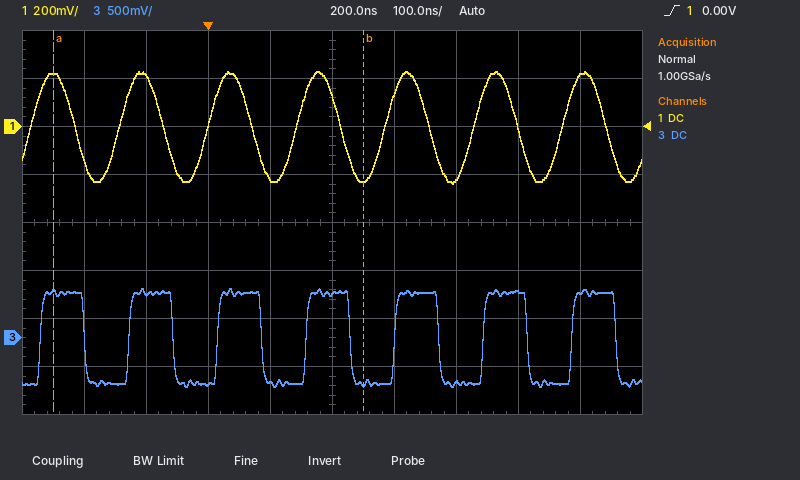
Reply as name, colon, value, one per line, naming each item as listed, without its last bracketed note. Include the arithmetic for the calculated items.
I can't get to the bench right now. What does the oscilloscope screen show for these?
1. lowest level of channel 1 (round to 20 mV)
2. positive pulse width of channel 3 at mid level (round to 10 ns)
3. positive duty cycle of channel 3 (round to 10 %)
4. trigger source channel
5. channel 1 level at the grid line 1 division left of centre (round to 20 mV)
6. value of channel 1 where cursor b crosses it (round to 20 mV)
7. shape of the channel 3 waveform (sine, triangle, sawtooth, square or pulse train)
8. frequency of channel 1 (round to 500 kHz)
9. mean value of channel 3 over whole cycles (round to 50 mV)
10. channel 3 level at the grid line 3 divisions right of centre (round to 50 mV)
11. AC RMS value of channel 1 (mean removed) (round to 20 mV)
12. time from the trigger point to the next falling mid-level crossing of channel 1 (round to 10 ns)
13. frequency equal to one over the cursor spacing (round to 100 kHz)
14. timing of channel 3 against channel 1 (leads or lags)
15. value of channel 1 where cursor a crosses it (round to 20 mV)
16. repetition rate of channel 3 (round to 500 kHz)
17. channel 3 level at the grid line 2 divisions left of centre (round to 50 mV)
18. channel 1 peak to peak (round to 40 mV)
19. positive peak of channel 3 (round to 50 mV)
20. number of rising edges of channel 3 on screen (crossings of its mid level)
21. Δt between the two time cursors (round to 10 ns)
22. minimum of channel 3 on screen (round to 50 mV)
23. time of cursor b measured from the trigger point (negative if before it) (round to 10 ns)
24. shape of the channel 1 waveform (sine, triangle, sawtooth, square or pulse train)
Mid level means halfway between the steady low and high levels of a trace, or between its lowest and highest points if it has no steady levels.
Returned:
lowest level of channel 1: -240 mV
positive pulse width of channel 3 at mid level: 70 ns
positive duty cycle of channel 3: 50 %
trigger source channel: channel 1
channel 1 level at the grid line 1 division left of centre: -220 mV
value of channel 1 where cursor b crosses it: -220 mV
shape of the channel 3 waveform: square
frequency of channel 1: 7.0 MHz
mean value of channel 3 over whole cycles: -500 mV + 0.5 × (500 mV − (-500 mV)) ≈ 0 mV
channel 3 level at the grid line 3 divisions right of centre: 500 mV
AC RMS value of channel 1 (mean removed): 480 mV / (2√2) ≈ 170 mV, so 160 mV to the nearest 20 mV
time from the trigger point to the next falling mid-level crossing of channel 1: 70 ns
frequency equal to one over the cursor spacing: 1 / 500 ns ≈ 2.0 MHz
timing of channel 3 against channel 1: lags
value of channel 1 where cursor a crosses it: 220 mV
repetition rate of channel 3: 7.0 MHz
channel 3 level at the grid line 2 divisions left of centre: -500 mV
channel 1 peak to peak: 480 mV
positive peak of channel 3: 500 mV
number of rising edges of channel 3 on screen: 7
Δt between the two time cursors: 500 ns
minimum of channel 3 on screen: -500 mV
time of cursor b measured from the trigger point (negative if before it): +250 ns
shape of the channel 1 waveform: sine
